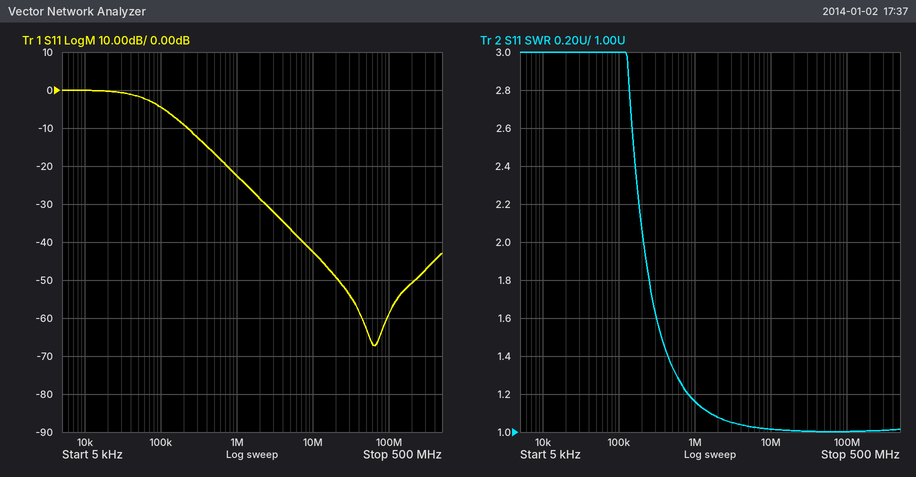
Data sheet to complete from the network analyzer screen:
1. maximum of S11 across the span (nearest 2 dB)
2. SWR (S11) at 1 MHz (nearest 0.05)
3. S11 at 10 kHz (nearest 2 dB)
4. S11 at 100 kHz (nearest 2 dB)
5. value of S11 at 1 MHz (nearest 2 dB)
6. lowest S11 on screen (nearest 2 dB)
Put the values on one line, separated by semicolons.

0 dB; 1.15; 0 dB; -4 dB; -22 dB; -68 dB
